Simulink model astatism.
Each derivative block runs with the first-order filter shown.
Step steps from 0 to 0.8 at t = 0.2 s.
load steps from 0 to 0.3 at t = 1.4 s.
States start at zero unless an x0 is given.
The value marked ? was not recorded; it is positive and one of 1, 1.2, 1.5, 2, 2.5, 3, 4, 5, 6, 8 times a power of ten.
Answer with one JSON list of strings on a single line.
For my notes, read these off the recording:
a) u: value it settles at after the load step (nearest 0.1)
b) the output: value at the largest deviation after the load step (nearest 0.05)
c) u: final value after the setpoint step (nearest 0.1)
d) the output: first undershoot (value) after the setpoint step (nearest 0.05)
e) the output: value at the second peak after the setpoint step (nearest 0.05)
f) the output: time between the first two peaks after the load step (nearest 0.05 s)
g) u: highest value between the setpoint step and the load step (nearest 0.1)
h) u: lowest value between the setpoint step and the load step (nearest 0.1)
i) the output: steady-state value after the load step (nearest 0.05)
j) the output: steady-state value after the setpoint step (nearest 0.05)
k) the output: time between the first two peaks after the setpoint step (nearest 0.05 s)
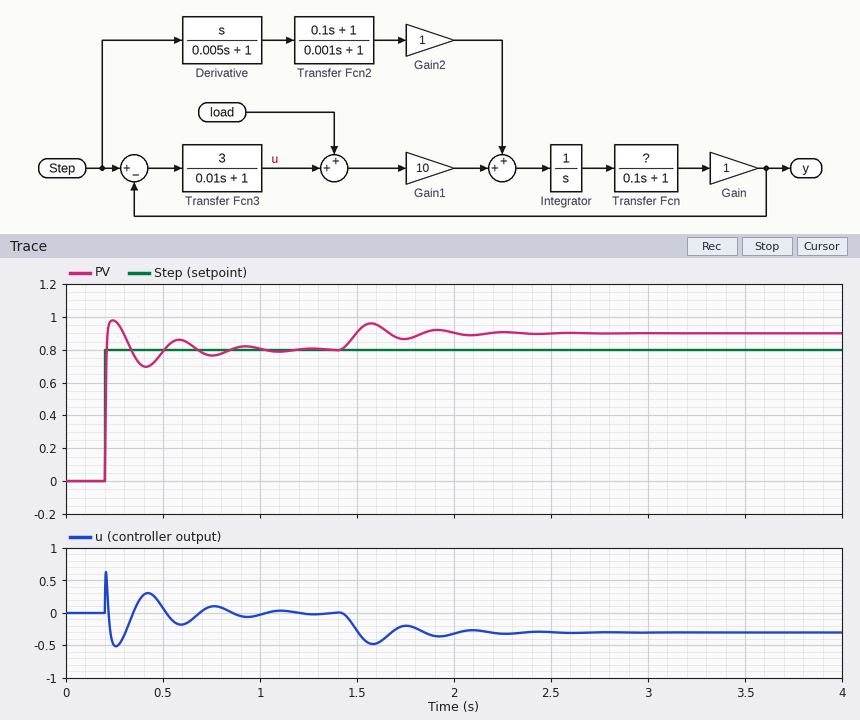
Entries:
["-0.3", "0.95", "0.0", "0.70", "0.85", "0.35 s", "0.6", "-0.5", "0.90", "0.80", "0.35 s"]
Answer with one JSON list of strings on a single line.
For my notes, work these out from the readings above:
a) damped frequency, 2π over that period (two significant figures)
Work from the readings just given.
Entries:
["18 rad/s"]
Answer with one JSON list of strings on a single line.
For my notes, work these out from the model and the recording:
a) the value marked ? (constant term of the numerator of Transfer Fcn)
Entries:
["1.2"]
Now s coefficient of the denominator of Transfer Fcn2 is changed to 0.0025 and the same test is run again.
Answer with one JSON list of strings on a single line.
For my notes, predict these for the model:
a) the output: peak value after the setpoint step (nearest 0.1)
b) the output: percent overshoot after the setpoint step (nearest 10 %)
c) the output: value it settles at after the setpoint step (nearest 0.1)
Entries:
["1.0", "20 %", "0.8"]
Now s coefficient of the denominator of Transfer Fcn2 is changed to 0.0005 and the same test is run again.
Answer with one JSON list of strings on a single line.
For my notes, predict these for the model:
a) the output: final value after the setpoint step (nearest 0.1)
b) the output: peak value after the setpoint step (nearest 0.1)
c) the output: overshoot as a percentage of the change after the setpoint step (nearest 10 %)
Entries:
["0.8", "1.0", "20 %"]
